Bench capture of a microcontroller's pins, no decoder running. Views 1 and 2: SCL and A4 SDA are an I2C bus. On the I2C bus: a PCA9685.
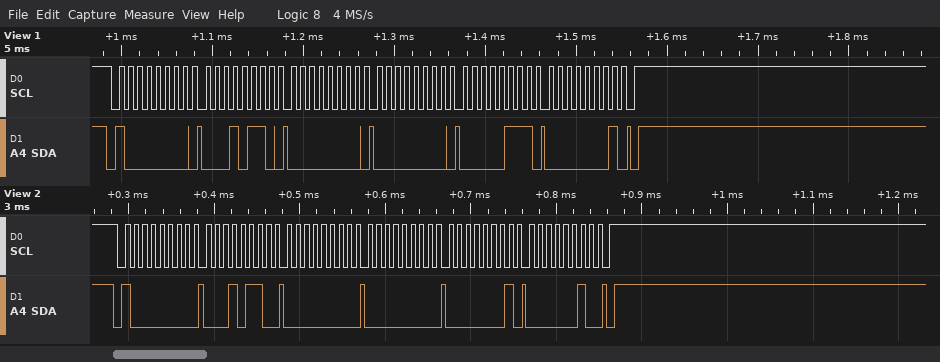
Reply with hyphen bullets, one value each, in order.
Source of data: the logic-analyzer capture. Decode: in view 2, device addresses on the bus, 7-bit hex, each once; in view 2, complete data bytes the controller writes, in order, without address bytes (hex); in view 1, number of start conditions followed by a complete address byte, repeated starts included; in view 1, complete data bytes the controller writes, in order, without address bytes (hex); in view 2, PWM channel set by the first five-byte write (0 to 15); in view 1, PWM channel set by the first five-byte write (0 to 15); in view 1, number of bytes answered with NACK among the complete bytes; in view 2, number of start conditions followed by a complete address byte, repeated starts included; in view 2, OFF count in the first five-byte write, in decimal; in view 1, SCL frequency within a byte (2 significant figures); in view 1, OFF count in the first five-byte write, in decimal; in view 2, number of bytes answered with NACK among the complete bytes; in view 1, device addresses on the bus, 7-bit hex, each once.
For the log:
- 0x40
- 16 00 00 01 02
- 1
- 16 00 00 07 01
- 4
- 4
- 0
- 1
- 513
- 100 kHz
- 263
- 0
- 0x40
